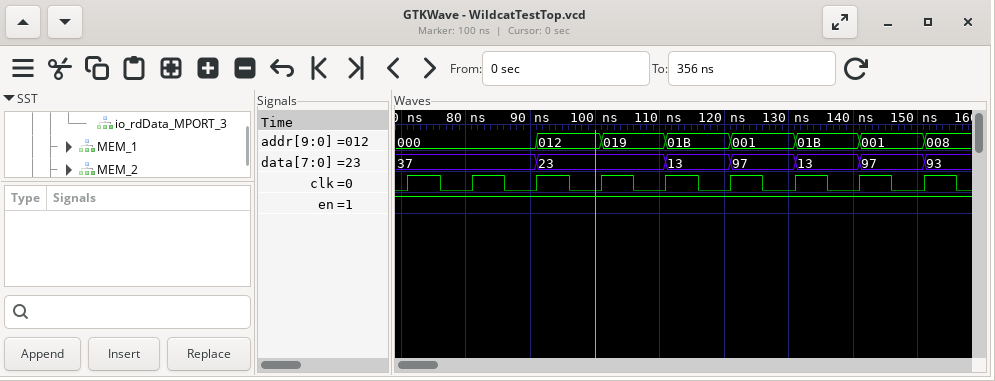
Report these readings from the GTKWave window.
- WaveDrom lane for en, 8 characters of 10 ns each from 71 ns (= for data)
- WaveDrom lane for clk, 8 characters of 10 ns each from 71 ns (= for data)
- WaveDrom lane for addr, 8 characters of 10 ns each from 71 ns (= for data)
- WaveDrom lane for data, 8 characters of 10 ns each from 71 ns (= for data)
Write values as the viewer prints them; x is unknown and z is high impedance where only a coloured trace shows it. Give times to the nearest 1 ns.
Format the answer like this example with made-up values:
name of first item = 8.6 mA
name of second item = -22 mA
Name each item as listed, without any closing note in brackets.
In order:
WaveDrom lane for en, 8 characters of 10 ns each from 71 ns = {name: 'en', wave: '1.......'}
WaveDrom lane for clk, 8 characters of 10 ns each from 71 ns = {name: 'clk', wave: 'p.......'}
WaveDrom lane for addr, 8 characters of 10 ns each from 71 ns = {name: 'addr', wave: '=.======', data: '000 012 019 01B 001 01B 001'}
WaveDrom lane for data, 8 characters of 10 ns each from 71 ns = {name: 'data', wave: '=.=.====', data: '37 23 13 97 13 97'}
